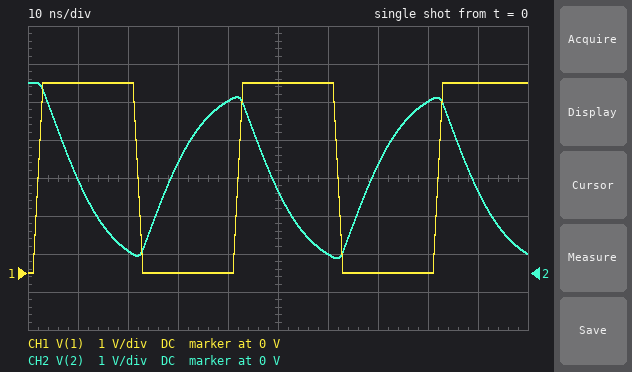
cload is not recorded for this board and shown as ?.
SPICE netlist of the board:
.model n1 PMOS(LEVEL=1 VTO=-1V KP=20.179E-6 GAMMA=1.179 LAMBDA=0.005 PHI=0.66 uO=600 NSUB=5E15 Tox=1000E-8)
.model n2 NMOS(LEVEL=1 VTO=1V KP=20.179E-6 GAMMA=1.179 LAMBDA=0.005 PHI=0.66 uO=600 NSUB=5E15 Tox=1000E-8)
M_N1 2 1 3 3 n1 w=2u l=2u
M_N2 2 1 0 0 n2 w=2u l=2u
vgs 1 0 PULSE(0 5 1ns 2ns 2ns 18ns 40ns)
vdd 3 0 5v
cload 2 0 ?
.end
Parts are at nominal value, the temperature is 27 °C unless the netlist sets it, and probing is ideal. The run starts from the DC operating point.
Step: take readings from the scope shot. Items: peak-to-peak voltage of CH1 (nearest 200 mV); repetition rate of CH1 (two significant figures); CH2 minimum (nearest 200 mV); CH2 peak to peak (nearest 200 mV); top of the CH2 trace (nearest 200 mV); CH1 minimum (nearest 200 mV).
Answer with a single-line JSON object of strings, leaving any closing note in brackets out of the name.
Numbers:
{"peak-to-peak voltage of CH1": "5.0 V", "repetition rate of CH1": "25 MHz", "CH2 minimum": "400 mV", "CH2 peak to peak": "4.6 V", "top of the CH2 trace": "5.0 V", "CH1 minimum": "0 V"}
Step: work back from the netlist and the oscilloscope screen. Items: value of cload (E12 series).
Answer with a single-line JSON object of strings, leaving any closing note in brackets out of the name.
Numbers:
{"value of cload": "470 fF"}
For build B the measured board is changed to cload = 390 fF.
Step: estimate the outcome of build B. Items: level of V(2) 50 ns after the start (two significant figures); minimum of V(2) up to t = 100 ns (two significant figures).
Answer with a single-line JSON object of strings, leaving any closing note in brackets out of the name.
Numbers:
{"level of V(2) 50 ns after the start": "1.9 V", "minimum of V(2) up to t = 100 ns": "220 mV"}
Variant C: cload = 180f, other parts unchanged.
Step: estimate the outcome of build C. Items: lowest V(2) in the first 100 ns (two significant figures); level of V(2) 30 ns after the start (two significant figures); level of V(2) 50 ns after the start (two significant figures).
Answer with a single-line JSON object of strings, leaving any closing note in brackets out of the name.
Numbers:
{"lowest V(2) in the first 100 ns": "2.6 mV", "level of V(2) 30 ns after the start": "4.6 V", "level of V(2) 50 ns after the start": "410 mV"}
